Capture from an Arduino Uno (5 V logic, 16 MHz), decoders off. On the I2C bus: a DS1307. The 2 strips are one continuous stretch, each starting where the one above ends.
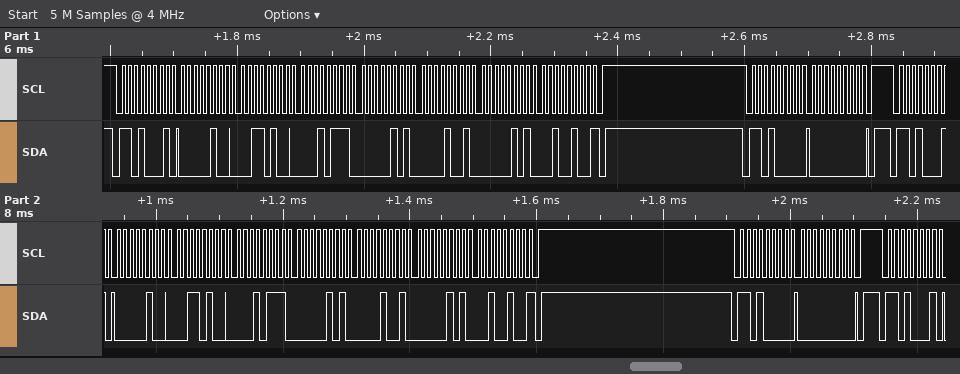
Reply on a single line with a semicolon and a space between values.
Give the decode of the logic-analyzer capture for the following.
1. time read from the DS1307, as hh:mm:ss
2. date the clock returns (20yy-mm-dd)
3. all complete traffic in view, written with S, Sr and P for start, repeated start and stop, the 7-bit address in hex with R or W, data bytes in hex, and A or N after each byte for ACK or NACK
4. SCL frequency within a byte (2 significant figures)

17:34:04; 2024-05-09; S 68R A 04 A 34 A 17 A 05 A 09 A 05 A 24 N P S 68W A 00 A P S 68R A 04 A 34 A 17 A 05 A 09 A 05 A 24 N P S 68W A 00 A P S 68R A; 100 kHz
